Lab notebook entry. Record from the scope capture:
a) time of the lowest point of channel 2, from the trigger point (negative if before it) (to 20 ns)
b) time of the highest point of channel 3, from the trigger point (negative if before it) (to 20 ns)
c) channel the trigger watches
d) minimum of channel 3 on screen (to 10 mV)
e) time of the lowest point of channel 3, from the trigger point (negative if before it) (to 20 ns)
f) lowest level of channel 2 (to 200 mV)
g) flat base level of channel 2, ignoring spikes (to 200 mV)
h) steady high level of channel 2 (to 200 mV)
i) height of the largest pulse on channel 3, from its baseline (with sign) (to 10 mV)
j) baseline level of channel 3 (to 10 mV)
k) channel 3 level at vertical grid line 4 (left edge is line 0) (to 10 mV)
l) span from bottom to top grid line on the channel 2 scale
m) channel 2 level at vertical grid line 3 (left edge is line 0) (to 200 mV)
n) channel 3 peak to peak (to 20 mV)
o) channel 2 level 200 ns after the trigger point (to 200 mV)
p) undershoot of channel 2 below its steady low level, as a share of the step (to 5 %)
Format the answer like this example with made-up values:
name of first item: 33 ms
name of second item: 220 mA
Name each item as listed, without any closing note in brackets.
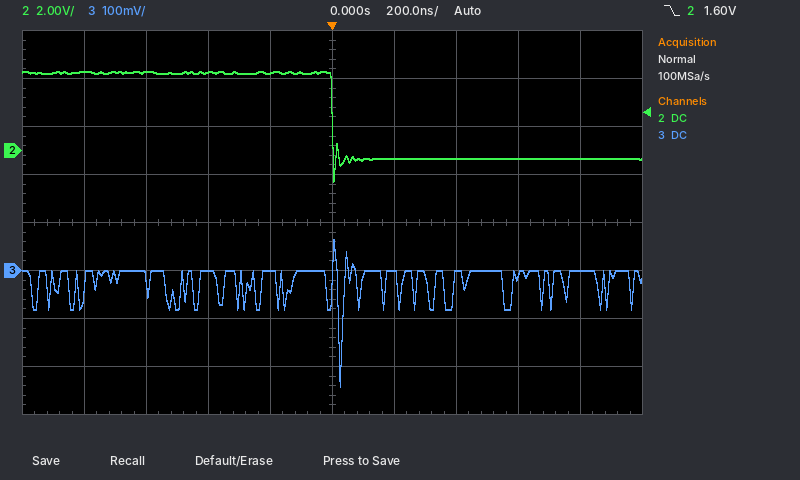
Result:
time of the lowest point of channel 2, from the trigger point (negative if before it): 0 ns
time of the highest point of channel 3, from the trigger point (negative if before it): 0 ns
channel the trigger watches: channel 2
minimum of channel 3 on screen: -240 mV
time of the lowest point of channel 3, from the trigger point (negative if before it): +20 ns
lowest level of channel 2: -1.2 V
flat base level of channel 2, ignoring spikes: -400 mV
steady high level of channel 2: 3.2 V
height of the largest pulse on channel 3, from its baseline (with sign): -240 mV
baseline level of channel 3: 0 mV
channel 3 level at vertical grid line 4 (left edge is line 0): 0 mV
span from bottom to top grid line on the channel 2 scale: 16 V
channel 2 level at vertical grid line 3 (left edge is line 0): 3.2 V
channel 3 peak to peak: 300 mV
channel 2 level 200 ns after the trigger point: -400 mV
undershoot of channel 2 below its steady low level, as a share of the step: 25 %
